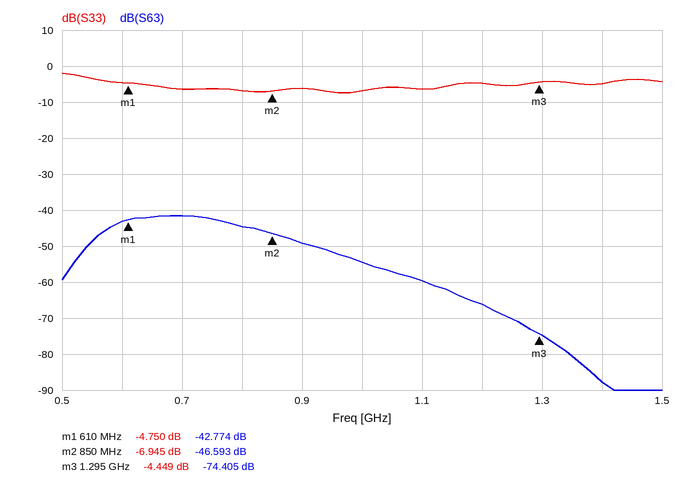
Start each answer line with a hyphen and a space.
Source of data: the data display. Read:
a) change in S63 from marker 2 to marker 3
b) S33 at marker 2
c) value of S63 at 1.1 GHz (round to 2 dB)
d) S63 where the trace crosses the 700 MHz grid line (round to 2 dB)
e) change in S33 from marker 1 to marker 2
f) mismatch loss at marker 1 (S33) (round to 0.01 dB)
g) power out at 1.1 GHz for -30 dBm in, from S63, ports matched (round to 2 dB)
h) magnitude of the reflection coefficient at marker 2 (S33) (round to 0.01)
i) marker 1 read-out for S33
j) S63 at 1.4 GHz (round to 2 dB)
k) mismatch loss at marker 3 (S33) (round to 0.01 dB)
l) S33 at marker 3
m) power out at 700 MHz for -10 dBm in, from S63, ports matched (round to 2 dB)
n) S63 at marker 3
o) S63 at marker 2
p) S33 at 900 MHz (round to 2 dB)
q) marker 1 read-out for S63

- -27.812 dB
- -6.945 dB
- -60 dB
- -42 dB
- -2.195 dB
- 1.77 dB
- -90 dBm
- 0.45
- -4.750 dB
- -88 dB
- 1.93 dB
- -4.449 dB
- -52 dBm
- -74.405 dB
- -46.593 dB
- -6 dB
- -42.774 dB
